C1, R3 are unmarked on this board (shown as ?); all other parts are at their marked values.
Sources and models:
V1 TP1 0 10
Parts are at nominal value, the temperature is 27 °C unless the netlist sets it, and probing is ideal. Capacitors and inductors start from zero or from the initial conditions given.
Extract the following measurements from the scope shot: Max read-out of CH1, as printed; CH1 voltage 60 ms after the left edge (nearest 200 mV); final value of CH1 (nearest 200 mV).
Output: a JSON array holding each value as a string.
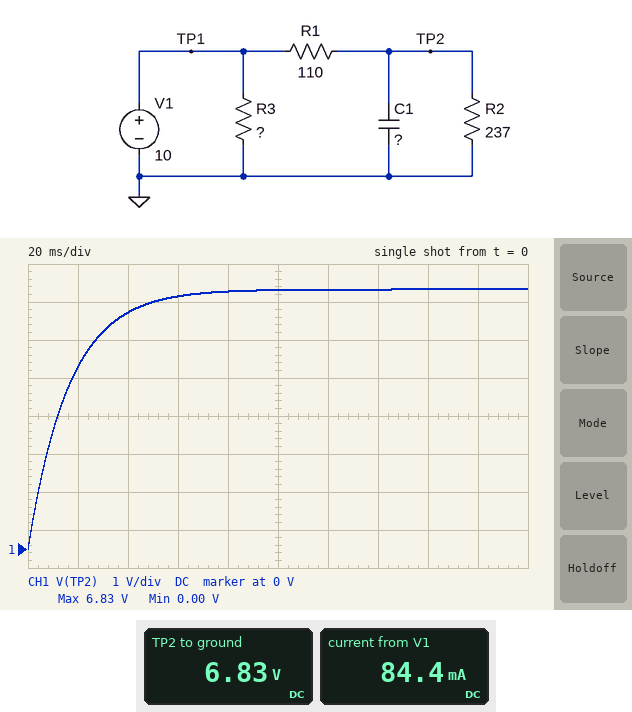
["6.83 V", "6.6 V", "6.8 V"]
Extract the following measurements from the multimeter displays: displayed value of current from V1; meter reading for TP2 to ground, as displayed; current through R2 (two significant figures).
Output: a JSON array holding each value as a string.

["84.4 mA", "6.83 V", "29 mA"]
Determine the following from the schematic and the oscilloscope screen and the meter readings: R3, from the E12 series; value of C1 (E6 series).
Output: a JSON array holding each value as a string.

["180 Ω", "220 µF"]
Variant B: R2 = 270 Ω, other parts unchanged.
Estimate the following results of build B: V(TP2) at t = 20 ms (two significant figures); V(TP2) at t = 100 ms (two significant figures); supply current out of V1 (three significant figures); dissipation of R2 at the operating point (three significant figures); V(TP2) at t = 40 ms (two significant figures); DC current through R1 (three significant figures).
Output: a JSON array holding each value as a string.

["4.9 V", "7.1 V", "81.9 mA", "187 mW", "6.4 V", "26.3 mA"]
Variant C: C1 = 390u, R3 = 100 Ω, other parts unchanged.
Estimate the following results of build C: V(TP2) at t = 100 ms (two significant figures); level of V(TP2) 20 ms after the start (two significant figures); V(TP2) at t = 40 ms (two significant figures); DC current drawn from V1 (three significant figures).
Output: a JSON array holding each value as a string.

["6.6 V", "3.4 V", "5.1 V", "129 mA"]
